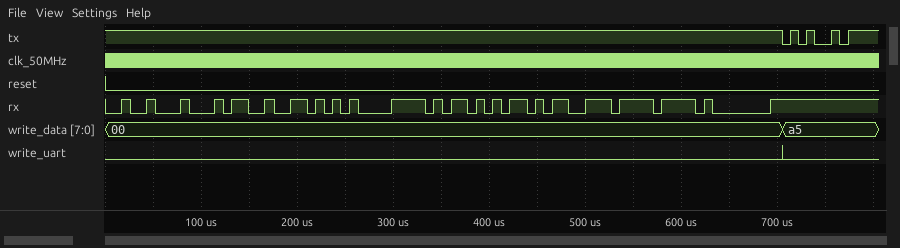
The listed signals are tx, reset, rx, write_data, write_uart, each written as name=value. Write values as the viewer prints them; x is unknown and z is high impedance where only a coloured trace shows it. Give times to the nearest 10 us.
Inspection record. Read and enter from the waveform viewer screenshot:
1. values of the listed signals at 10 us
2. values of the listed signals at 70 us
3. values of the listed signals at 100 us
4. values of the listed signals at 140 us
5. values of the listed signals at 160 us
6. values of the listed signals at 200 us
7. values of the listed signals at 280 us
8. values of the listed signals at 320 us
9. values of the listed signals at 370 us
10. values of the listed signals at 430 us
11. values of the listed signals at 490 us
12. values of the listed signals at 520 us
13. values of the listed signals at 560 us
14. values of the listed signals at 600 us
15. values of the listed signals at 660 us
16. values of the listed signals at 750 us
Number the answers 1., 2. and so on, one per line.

1. tx=1, reset=0, rx=0, write_data=00, write_uart=0
2. tx=1, reset=0, rx=0, write_data=00, write_uart=0
3. tx=1, reset=0, rx=0, write_data=00, write_uart=0
4. tx=1, reset=0, rx=1, write_data=00, write_uart=0
5. tx=1, reset=0, rx=0, write_data=00, write_uart=0
6. tx=1, reset=0, rx=1, write_data=00, write_uart=0
7. tx=1, reset=0, rx=0, write_data=00, write_uart=0
8. tx=1, reset=0, rx=1, write_data=00, write_uart=0
9. tx=1, reset=0, rx=1, write_data=00, write_uart=0
10. tx=1, reset=0, rx=1, write_data=00, write_uart=0
11. tx=1, reset=0, rx=0, write_data=00, write_uart=0
12. tx=1, reset=0, rx=1, write_data=00, write_uart=0
13. tx=1, reset=0, rx=1, write_data=00, write_uart=0
14. tx=1, reset=0, rx=1, write_data=00, write_uart=0
15. tx=1, reset=0, rx=0, write_data=00, write_uart=0
16. tx=0, reset=0, rx=1, write_data=a5, write_uart=0
